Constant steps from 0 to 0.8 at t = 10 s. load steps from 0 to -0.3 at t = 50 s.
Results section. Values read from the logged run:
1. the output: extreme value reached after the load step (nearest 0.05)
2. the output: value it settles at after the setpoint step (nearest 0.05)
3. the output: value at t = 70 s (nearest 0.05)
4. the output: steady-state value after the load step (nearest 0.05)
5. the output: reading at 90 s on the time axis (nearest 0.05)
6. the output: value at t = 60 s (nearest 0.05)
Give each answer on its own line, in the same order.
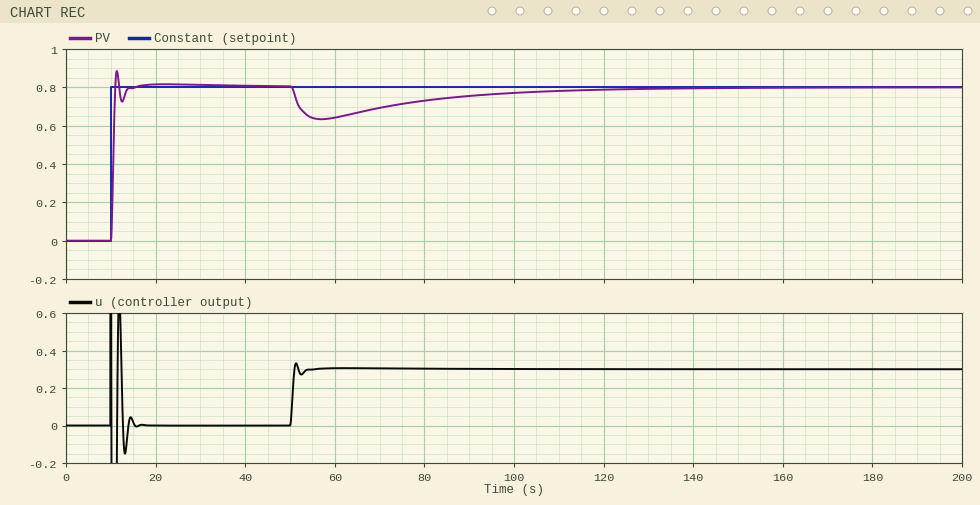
0.65
0.80
0.70
0.80
0.75
0.65
